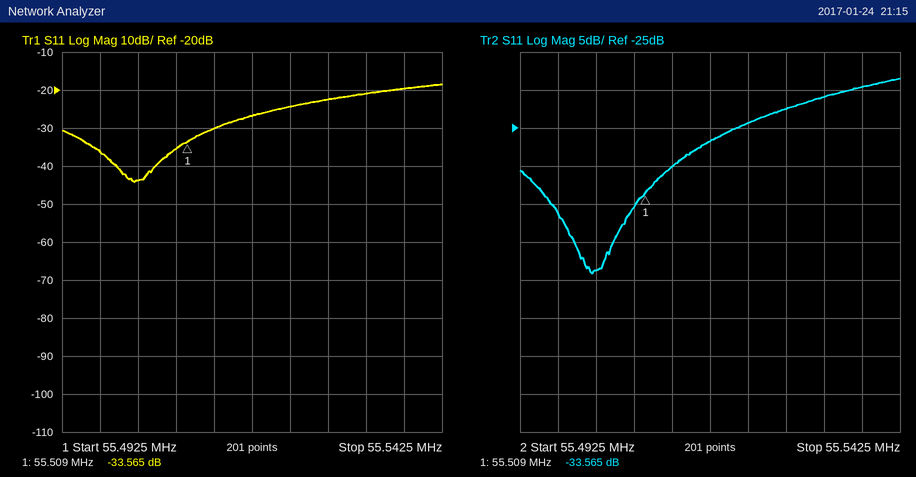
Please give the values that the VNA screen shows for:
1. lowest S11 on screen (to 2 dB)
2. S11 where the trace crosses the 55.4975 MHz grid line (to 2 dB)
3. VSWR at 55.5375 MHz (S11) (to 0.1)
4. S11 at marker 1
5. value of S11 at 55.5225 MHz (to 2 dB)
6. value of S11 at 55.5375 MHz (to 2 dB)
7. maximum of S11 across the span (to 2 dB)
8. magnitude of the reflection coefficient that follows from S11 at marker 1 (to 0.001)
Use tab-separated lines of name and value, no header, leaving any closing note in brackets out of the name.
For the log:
lowest S11 on screen	-44 dB
S11 where the trace crosses the 55.4975 MHz grid line	-36 dB
VSWR at 55.5375 MHz (S11)	1.2
S11 at marker 1	-33.565 dB
value of S11 at 55.5225 MHz	-24 dB
value of S11 at 55.5375 MHz	-20 dB
maximum of S11 across the span	-18 dB
magnitude of the reflection coefficient that follows from S11 at marker 1	0.021
